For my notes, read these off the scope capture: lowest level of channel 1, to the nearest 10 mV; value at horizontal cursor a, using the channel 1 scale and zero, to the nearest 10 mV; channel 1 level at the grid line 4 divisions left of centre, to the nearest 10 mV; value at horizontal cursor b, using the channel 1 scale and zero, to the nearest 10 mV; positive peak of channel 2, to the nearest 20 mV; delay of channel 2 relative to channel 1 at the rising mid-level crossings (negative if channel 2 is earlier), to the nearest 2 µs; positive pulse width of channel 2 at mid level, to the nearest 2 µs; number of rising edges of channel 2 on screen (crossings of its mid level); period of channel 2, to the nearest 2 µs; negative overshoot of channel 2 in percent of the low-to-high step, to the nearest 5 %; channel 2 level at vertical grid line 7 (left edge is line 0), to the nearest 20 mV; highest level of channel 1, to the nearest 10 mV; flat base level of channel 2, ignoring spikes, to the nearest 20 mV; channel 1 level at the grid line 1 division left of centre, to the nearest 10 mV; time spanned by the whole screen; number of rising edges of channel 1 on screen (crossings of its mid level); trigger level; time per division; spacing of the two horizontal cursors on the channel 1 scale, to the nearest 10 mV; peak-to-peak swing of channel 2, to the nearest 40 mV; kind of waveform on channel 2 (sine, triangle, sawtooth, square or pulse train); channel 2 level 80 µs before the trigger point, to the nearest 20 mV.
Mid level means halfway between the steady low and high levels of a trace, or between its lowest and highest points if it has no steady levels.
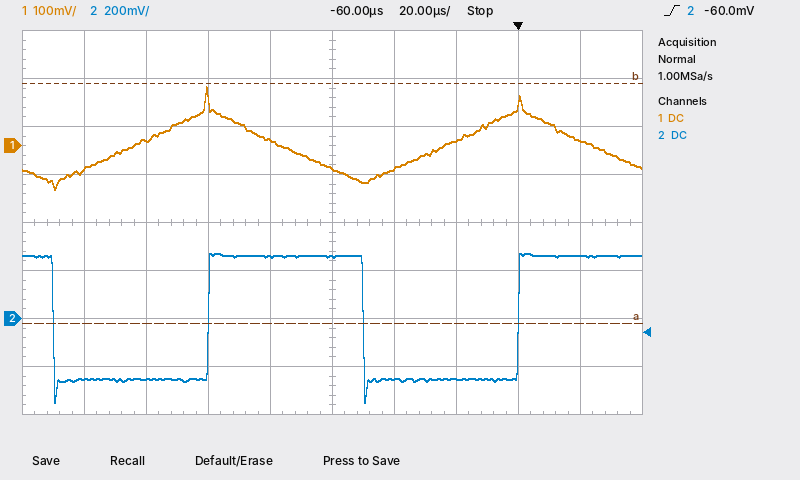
-90 mV
-370 mV
-50 mV
130 mV
280 mV
+18 µs
50 µs
2
100 µs
20 %
-260 mV
120 mV
-260 mV
10 mV
200 µs
2
-60.0 mV
20 µs
500 mV
640 mV
square
260 mV
